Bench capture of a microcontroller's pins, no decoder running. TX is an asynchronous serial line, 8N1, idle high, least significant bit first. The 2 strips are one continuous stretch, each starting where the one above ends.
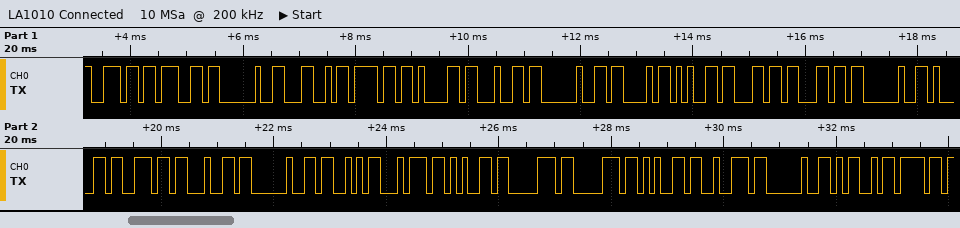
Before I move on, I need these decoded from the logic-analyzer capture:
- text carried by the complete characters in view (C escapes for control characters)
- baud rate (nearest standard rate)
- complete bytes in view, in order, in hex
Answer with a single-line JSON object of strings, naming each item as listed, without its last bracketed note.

{"text carried by the complete characters in view": "\"ng Load Cell and Stepper Mo\"", "baud rate": "9600 baud", "complete bytes in view, in order, in hex": "6E 67 20 4C 6F 61 64 20 43 65 6C 6C 20 61 6E 64 20 53 74 65 70 70 65 72 20 4D 6F"}
